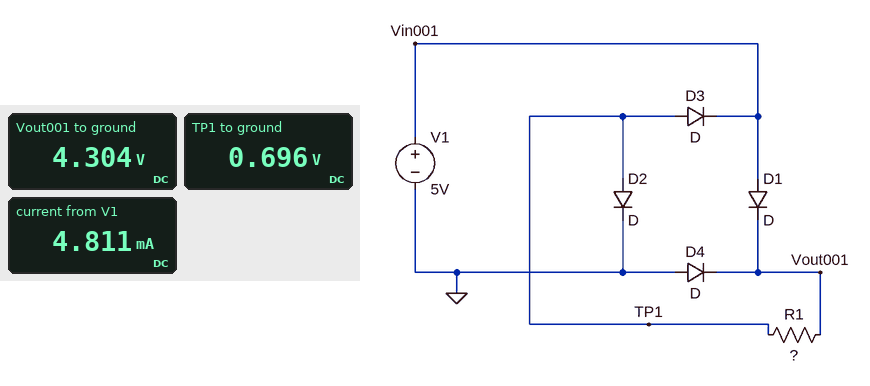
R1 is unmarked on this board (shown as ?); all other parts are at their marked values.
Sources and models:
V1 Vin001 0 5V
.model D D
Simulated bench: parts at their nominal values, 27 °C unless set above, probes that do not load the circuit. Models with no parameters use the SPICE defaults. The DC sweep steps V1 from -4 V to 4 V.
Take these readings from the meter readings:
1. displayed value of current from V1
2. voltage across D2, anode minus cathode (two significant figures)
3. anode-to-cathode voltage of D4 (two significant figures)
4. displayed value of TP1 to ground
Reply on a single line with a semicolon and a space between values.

4.811 mA; 700 mV; -4.3 V; 0.696 V
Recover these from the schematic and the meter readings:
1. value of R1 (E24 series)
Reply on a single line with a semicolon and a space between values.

750 Ω
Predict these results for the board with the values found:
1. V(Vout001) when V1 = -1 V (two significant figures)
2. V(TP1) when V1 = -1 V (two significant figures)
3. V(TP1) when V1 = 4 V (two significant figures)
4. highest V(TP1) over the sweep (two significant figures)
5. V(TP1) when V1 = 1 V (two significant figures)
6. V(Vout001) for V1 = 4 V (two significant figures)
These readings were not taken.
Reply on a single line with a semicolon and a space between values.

-500 mV; -500 mV; 690 mV; 690 mV; 500 mV; 3.3 V
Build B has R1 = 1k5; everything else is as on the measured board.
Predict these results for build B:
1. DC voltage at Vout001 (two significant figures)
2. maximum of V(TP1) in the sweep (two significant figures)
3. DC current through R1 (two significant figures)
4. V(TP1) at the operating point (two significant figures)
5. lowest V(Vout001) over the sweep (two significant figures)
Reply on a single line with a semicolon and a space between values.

4.3 V; 670 mV; 2.4 mA; 680 mV; -670 mV
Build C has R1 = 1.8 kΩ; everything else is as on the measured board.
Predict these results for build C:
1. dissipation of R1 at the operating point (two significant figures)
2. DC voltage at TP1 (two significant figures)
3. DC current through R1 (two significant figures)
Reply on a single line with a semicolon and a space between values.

7.4 mW; 670 mV; 2.0 mA
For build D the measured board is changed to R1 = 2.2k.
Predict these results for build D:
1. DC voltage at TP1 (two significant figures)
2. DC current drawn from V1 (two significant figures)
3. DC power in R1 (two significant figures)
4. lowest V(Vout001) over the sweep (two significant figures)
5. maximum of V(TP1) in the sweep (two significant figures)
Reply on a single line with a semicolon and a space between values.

670 mV; 1.7 mA; 6.1 mW; -660 mV; 660 mV
